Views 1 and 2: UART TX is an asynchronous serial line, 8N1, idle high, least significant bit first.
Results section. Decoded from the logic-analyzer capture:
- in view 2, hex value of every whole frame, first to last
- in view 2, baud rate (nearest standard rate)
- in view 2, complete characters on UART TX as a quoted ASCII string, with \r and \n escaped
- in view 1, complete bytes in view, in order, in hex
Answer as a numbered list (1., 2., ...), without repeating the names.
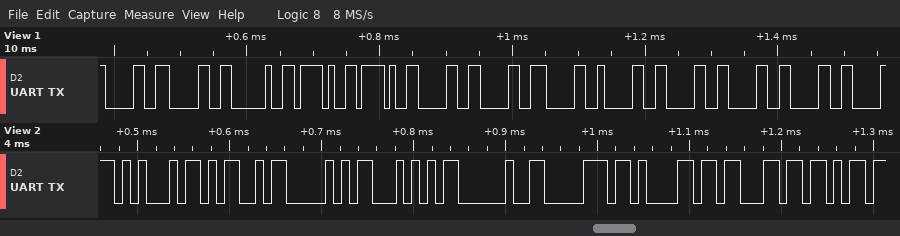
1. 45 4D 50 54 20 70 61 63 6B
2. 115200 baud
3. "EMPT pack"
4. 30 30 20 2F 2F 30 30 30 30 30 30 30
